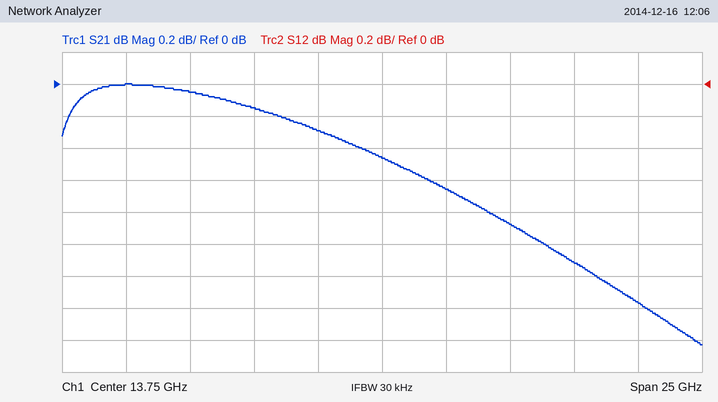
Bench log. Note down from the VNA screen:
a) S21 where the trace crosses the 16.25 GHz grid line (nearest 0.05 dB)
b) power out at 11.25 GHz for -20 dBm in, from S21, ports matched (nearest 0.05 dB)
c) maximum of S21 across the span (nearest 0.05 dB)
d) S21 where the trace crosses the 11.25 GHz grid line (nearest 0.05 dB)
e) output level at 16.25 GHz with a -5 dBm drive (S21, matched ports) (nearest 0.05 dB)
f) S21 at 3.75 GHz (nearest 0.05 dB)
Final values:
-0.65 dB
-20.30 dBm
0.00 dB
-0.30 dB
-5.65 dBm
0.00 dB
